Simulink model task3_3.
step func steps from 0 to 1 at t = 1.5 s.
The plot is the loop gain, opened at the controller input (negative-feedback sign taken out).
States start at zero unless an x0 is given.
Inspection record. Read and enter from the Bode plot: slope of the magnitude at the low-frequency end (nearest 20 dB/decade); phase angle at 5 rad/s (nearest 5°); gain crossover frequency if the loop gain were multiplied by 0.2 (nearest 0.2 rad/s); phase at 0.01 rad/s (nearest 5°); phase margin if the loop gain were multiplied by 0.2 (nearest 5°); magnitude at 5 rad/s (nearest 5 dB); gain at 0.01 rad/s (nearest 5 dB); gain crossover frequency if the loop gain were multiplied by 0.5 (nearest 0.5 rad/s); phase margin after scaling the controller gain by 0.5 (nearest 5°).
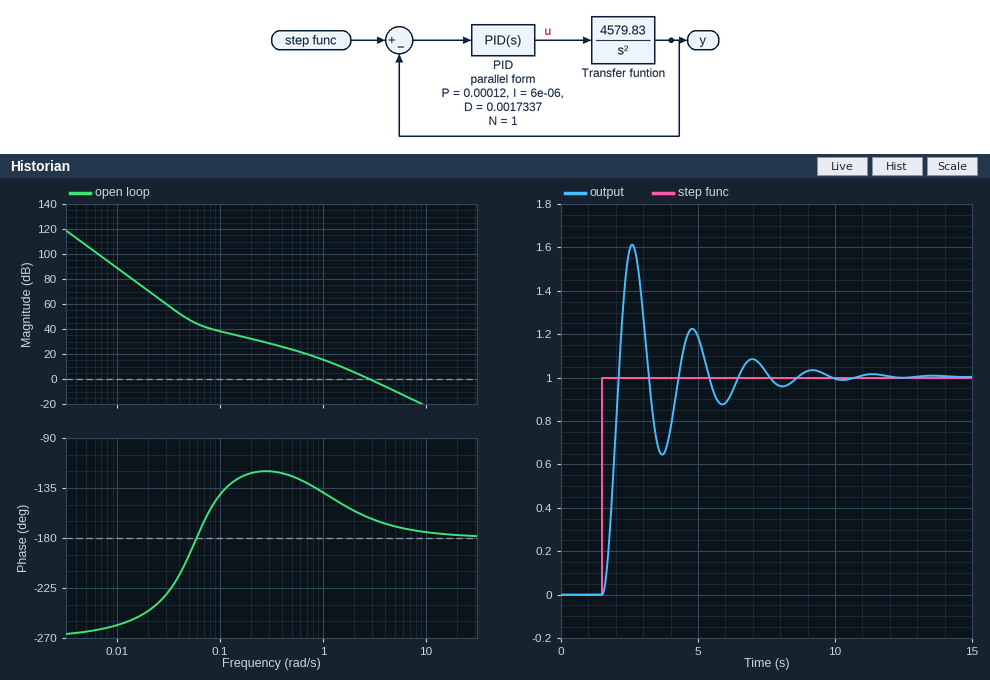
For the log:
-60 dB/decade
-170°
1.2 rad/s
-260°
40°
-10 dB
90 dB
2.0 rad/s
25°
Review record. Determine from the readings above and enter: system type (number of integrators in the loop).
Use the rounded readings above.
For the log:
3
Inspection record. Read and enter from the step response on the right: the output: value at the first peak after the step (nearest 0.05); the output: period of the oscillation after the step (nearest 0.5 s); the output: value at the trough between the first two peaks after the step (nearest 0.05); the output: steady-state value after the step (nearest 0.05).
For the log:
1.60
2.0 s
0.65
1.00
